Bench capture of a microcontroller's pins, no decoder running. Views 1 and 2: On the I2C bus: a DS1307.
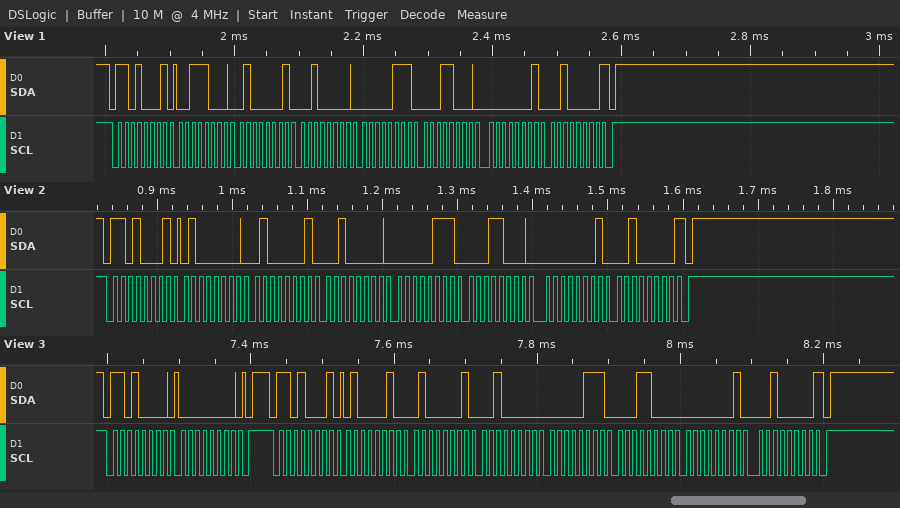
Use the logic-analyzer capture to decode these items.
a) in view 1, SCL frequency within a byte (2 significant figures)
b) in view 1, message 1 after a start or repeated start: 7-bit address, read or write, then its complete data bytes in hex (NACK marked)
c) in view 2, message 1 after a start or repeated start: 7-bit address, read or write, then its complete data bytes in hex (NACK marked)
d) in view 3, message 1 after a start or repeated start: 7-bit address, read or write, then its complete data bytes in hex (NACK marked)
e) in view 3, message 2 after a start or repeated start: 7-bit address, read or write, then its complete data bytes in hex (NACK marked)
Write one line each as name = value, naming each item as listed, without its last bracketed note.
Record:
in view 1, SCL frequency within a byte = 100 kHz
in view 1, message 1 after a start or repeated start: 7-bit address, read or write, then its complete data bytes in hex = 0x68 read: 38 41 20 07 18 01 20 NACK
in view 2, message 1 after a start or repeated start: 7-bit address, read or write, then its complete data bytes in hex = 0x68 read: 40 41 20 07 18 01 20 NACK
in view 3, message 1 after a start or repeated start: 7-bit address, read or write, then its complete data bytes in hex = 0x68 write: 00
in view 3, message 2 after a start or repeated start: 7-bit address, read or write, then its complete data bytes in hex = 0x68 read: 42 41 20 07 18 01 20 NACK
